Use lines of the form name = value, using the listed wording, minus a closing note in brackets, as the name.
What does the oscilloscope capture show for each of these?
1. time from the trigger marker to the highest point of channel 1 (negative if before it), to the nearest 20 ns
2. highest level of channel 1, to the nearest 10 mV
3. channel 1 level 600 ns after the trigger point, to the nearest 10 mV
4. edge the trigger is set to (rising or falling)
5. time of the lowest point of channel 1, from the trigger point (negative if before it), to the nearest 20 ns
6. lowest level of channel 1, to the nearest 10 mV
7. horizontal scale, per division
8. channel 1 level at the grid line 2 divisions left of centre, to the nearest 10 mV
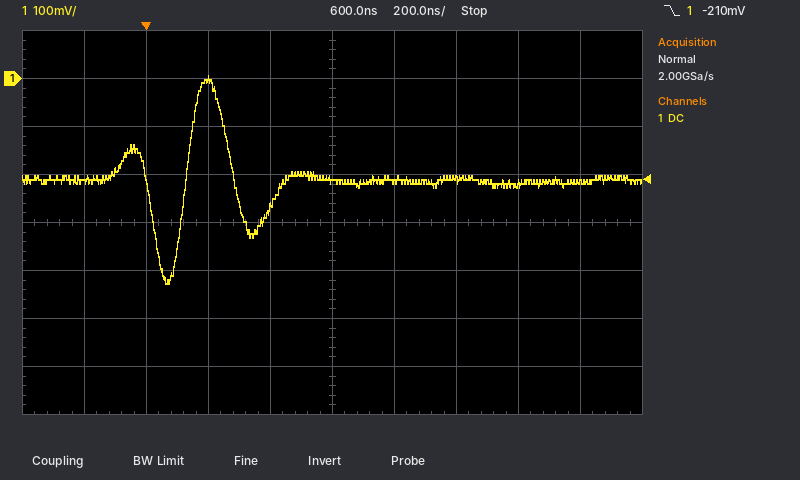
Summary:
time from the trigger marker to the highest point of channel 1 (negative if before it), to the nearest 20 ns = +200 ns
highest level of channel 1, to the nearest 10 mV = 10 mV
channel 1 level 600 ns after the trigger point, to the nearest 10 mV = -210 mV
edge the trigger is set to = falling
time of the lowest point of channel 1, from the trigger point (negative if before it), to the nearest 20 ns = +60 ns
lowest level of channel 1, to the nearest 10 mV = -430 mV
horizontal scale, per division = 200 ns
channel 1 level at the grid line 2 divisions left of centre, to the nearest 10 mV = 0 mV
